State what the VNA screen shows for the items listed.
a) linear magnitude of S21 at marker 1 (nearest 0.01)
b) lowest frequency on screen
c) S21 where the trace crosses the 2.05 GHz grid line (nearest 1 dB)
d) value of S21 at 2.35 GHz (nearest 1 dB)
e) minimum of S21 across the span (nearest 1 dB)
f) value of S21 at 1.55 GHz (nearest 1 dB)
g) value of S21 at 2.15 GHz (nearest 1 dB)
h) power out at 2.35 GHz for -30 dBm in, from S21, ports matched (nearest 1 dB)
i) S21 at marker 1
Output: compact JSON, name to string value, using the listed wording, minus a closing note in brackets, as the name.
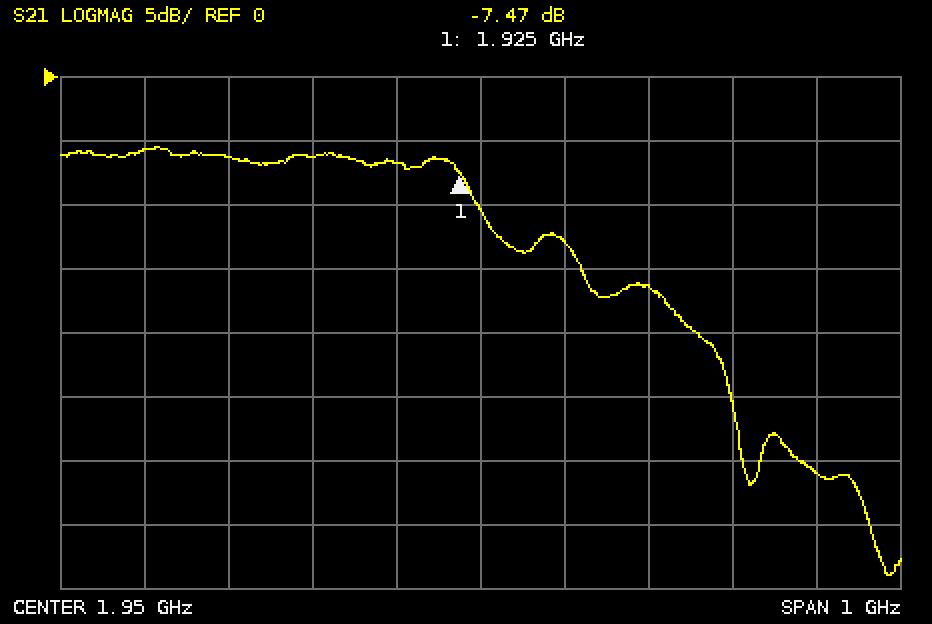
{"linear magnitude of S21 at marker 1": "0.42", "lowest frequency on screen": "1.45 GHz", "S21 where the trace crosses the 2.05 GHz grid line": "-13 dB", "value of S21 at 2.35 GHz": "-31 dB", "minimum of S21 across the span": "-39 dB", "value of S21 at 1.55 GHz": "-6 dB", "value of S21 at 2.15 GHz": "-16 dB", "power out at 2.35 GHz for -30 dBm in, from S21, ports matched": "-61 dBm", "S21 at marker 1": "-7.47 dB"}
